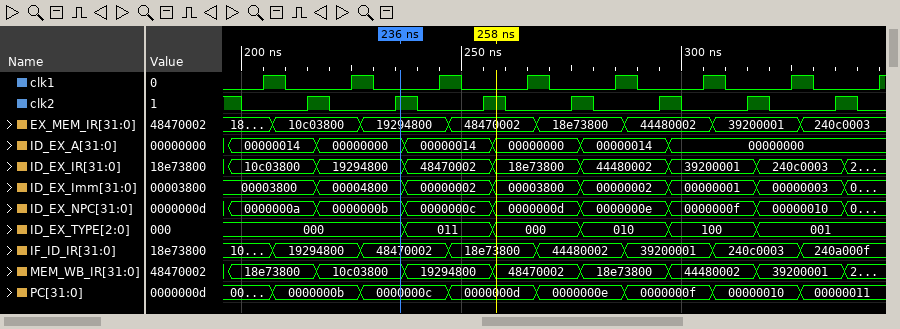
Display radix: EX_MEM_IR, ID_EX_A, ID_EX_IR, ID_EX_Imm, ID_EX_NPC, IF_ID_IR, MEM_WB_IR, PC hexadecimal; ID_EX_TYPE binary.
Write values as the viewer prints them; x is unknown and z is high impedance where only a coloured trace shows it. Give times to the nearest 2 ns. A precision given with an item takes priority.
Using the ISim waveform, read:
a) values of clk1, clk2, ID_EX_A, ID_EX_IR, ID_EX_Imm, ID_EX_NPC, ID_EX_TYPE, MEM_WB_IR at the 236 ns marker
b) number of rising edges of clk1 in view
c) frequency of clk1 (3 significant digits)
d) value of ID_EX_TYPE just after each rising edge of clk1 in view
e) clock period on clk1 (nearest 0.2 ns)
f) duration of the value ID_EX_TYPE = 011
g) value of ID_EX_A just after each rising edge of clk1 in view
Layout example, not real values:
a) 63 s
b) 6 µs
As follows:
a) clk1=0, clk2=1, ID_EX_A=00000000, ID_EX_IR=19294800, ID_EX_Imm=00004800, ID_EX_NPC=0000000b, ID_EX_TYPE=000, MEM_WB_IR=10c03800
b) 8
c) 50.0 MHz
d) 000, 000, 011, 000, 010, 100, 001, 001
e) 20 ns
f) 20 ns
g) 00000014, 00000000, 00000014, 00000000, 00000014, 00000000, 00000000, 00000000
